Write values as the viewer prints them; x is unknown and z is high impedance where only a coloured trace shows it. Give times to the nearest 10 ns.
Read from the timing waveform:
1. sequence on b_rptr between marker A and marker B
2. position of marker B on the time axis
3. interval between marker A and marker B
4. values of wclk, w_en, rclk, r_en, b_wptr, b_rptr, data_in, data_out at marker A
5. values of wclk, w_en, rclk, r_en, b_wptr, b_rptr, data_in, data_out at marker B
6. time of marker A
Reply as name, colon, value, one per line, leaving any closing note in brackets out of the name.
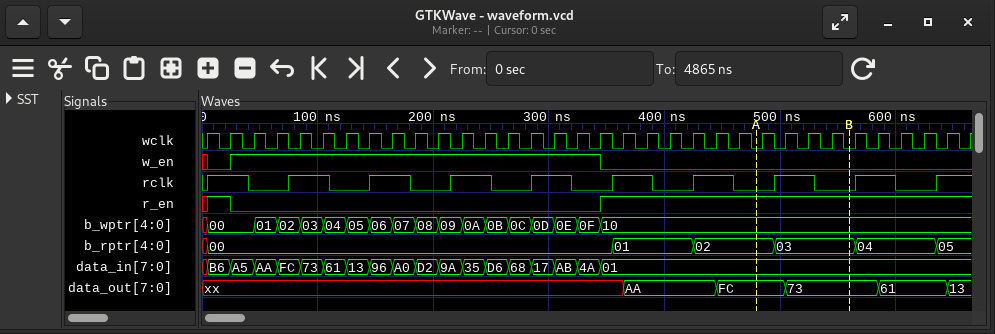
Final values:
sequence on b_rptr between marker A and marker B: 02, 03
position of marker B on the time axis: 560 ns
interval between marker A and marker B: 80 ns
values of wclk, w_en, rclk, r_en, b_wptr, b_rptr, data_in, data_out at marker A: wclk=0, w_en=0, rclk=0, r_en=1, b_wptr=10, b_rptr=02, data_in=01, data_out=FC
values of wclk, w_en, rclk, r_en, b_wptr, b_rptr, data_in, data_out at marker B: wclk=0, w_en=0, rclk=0, r_en=1, b_wptr=10, b_rptr=03, data_in=01, data_out=73
time of marker A: 480 ns
